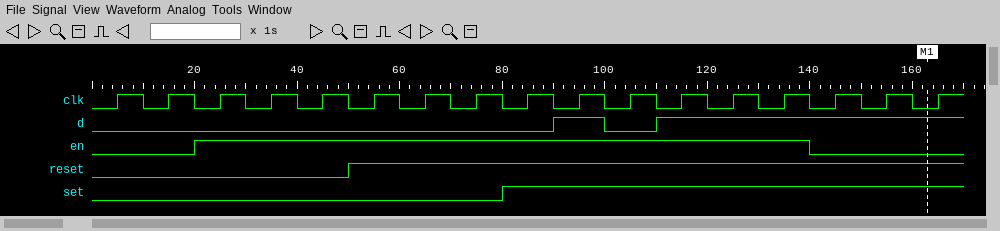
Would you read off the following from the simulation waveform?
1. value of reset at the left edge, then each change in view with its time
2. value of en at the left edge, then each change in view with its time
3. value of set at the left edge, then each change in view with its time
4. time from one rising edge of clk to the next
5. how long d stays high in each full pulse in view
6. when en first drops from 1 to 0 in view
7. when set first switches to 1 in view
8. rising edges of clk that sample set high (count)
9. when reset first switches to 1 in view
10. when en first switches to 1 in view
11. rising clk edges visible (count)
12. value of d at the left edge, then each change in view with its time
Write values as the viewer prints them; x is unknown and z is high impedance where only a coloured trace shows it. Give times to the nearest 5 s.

0, 1 at 50 s
0, 1 at 20 s, 0 at 140 s
0, 1 at 80 s
10 s
10 s
140 s
80 s
9
50 s
20 s
17
0, 1 at 90 s, 0 at 100 s, 1 at 110 s
